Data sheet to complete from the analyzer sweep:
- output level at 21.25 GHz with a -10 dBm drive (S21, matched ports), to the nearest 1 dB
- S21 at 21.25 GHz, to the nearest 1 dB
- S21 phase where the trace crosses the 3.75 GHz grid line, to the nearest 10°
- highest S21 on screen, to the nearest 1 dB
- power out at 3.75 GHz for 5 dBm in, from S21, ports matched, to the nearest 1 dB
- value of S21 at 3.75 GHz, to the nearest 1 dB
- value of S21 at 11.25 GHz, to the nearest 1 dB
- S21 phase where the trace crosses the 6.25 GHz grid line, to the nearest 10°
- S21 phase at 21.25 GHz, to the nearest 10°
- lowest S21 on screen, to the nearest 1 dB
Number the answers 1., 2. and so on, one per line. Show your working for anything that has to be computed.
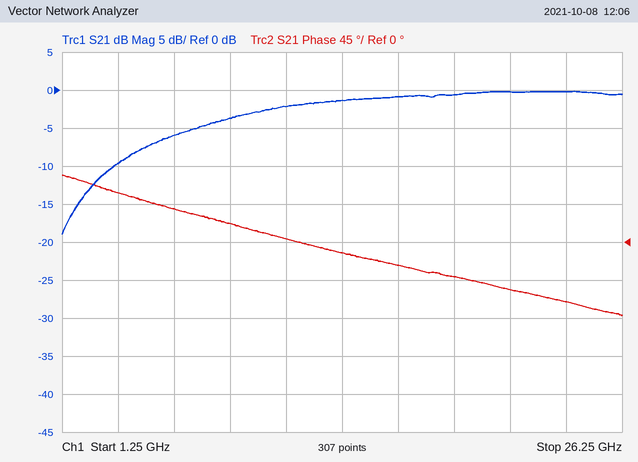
1. -10 dBm + (0 dB) = -10 dBm
2. 0 dB
3. 60°
4. 0 dB
5. 5 dBm + (-10 dB) = -5 dBm
6. -10 dB
7. -2 dB
8. 40°
9. -60°
10. -19 dB
